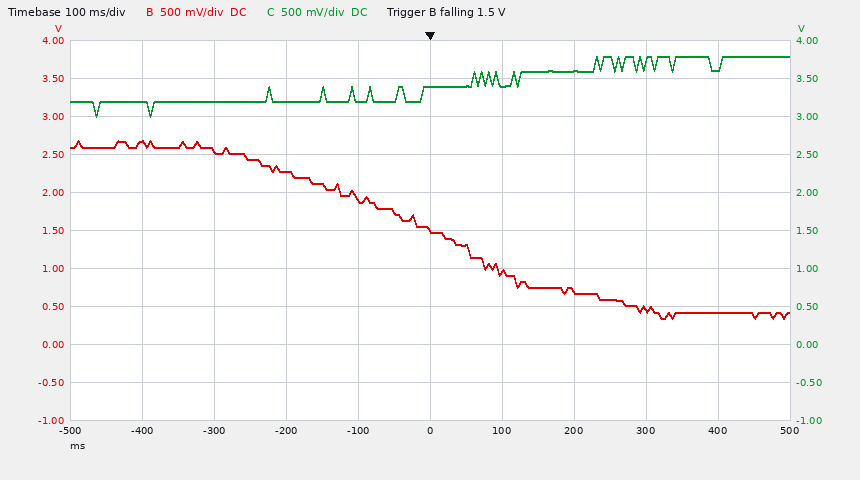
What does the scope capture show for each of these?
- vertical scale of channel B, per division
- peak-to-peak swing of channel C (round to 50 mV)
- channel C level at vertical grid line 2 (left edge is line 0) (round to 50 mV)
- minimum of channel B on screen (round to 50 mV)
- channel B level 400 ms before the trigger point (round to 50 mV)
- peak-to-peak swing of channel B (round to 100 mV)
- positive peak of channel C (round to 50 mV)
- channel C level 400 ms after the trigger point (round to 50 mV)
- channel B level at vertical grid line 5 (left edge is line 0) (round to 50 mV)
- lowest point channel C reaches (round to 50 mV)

500 mV
800 mV
3.20 V
350 mV
2.65 V
2.30 V
3.80 V
3.65 V
1.50 V
3.00 V
